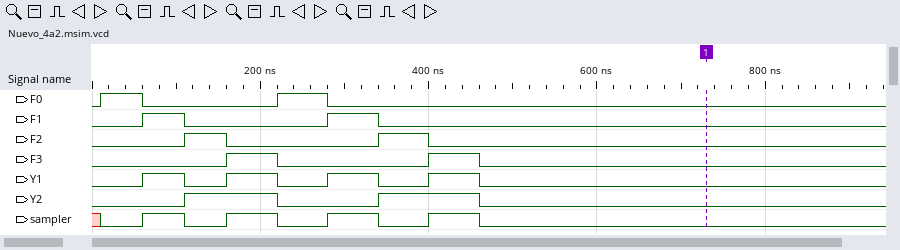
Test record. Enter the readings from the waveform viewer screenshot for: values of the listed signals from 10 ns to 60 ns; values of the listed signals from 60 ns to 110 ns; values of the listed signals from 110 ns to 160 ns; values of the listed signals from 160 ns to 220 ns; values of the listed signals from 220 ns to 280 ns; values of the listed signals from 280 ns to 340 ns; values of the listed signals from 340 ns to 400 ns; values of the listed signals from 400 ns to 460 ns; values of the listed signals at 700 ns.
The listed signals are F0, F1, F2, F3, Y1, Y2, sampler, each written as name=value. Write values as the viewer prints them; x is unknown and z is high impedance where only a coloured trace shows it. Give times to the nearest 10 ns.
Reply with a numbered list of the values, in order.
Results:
1. F0=1, F1=0, F2=0, F3=0, Y1=0, Y2=0, sampler=0
2. F0=0, F1=1, F2=0, F3=0, Y1=1, Y2=0, sampler=1
3. F0=0, F1=0, F2=1, F3=0, Y1=0, Y2=1, sampler=0
4. F0=0, F1=0, F2=0, F3=1, Y1=1, Y2=1, sampler=1
5. F0=1, F1=0, F2=0, F3=0, Y1=0, Y2=0, sampler=0
6. F0=0, F1=1, F2=0, F3=0, Y1=1, Y2=0, sampler=1
7. F0=0, F1=0, F2=1, F3=0, Y1=0, Y2=1, sampler=0
8. F0=0, F1=0, F2=0, F3=1, Y1=1, Y2=1, sampler=1
9. F0=0, F1=0, F2=0, F3=0, Y1=0, Y2=0, sampler=0
